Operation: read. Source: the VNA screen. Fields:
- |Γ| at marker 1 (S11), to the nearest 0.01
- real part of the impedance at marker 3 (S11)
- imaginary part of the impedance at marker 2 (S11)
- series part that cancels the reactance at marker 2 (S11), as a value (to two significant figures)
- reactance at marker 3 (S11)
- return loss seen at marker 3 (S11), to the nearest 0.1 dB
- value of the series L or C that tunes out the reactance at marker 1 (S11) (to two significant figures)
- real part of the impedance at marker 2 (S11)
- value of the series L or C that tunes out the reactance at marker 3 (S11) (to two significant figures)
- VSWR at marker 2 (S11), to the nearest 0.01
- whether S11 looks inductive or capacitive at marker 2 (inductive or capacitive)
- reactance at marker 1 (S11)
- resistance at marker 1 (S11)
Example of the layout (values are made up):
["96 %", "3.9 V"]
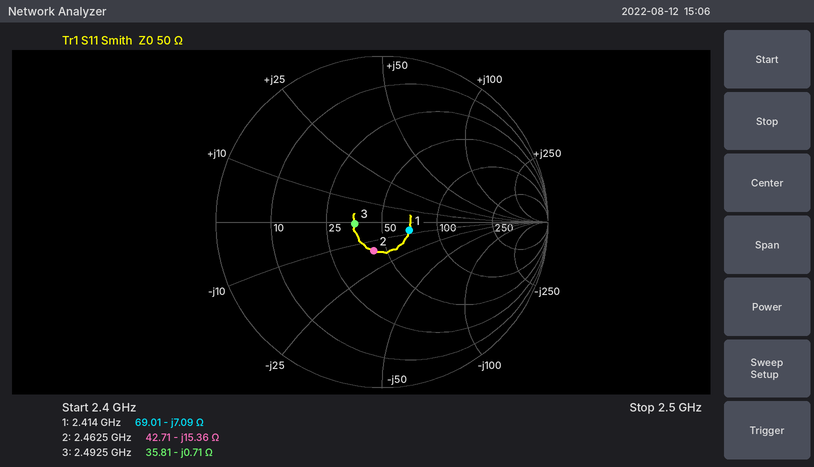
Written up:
["0.17", "35.81 Ω", "-15.36 Ω", "990 pH", "-0.71 Ω", "15.6 dB", "470 pH", "42.71 Ω", "45 pH", "1.44", "capacitive", "-7.09 Ω", "69.01 Ω"]
